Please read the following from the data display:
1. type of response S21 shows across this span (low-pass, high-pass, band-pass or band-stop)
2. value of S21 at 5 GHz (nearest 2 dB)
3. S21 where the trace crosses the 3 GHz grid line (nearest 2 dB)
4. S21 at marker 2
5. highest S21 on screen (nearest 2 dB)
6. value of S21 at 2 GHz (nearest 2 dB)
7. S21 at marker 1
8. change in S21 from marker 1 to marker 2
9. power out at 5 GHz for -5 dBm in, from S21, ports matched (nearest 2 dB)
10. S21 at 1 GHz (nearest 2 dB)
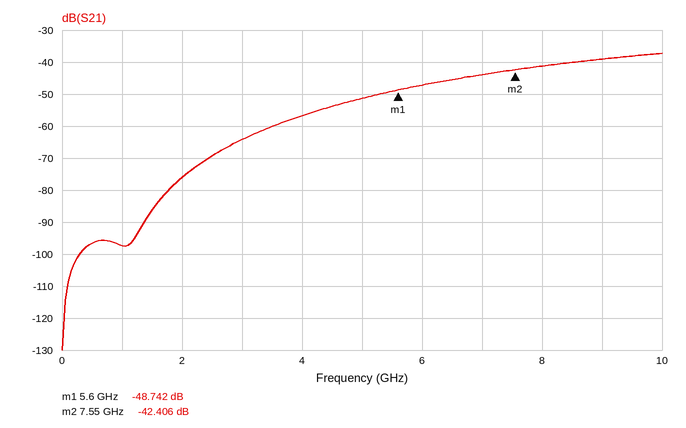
high-pass
-52 dB
-64 dB
-42.406 dB
-38 dB
-76 dB
-48.742 dB
6.336 dB
-56 dBm
-98 dB
